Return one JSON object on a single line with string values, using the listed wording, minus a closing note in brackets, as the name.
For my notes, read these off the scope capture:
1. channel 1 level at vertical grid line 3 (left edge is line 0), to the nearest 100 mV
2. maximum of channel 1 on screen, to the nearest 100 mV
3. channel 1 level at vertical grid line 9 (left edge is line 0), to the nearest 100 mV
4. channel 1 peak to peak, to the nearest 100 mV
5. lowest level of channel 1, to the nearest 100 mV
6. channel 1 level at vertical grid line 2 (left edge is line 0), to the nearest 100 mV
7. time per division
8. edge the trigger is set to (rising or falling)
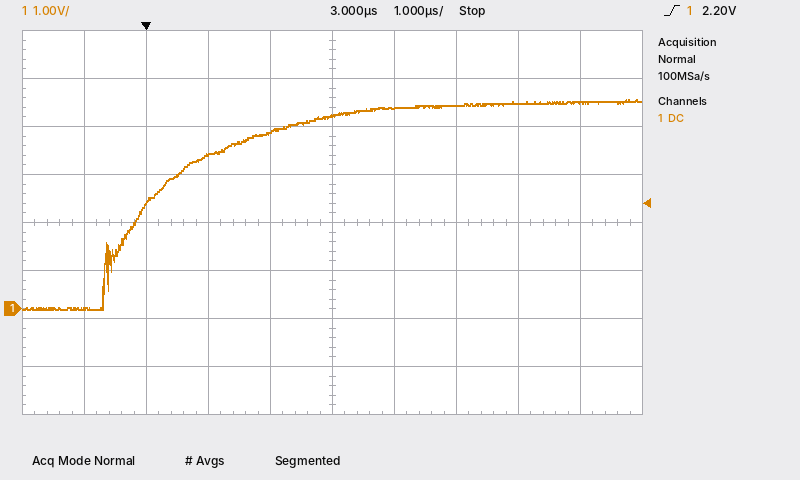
{"channel 1 level at vertical grid line 3 (left edge is line 0), to the nearest 100 mV": "3.2 V", "maximum of channel 1 on screen, to the nearest 100 mV": "4.4 V", "channel 1 level at vertical grid line 9 (left edge is line 0), to the nearest 100 mV": "4.3 V", "channel 1 peak to peak, to the nearest 100 mV": "4.4 V", "lowest level of channel 1, to the nearest 100 mV": "0.0 V", "channel 1 level at vertical grid line 2 (left edge is line 0), to the nearest 100 mV": "2.2 V", "time per division": "1 µs", "edge the trigger is set to": "rising"}
